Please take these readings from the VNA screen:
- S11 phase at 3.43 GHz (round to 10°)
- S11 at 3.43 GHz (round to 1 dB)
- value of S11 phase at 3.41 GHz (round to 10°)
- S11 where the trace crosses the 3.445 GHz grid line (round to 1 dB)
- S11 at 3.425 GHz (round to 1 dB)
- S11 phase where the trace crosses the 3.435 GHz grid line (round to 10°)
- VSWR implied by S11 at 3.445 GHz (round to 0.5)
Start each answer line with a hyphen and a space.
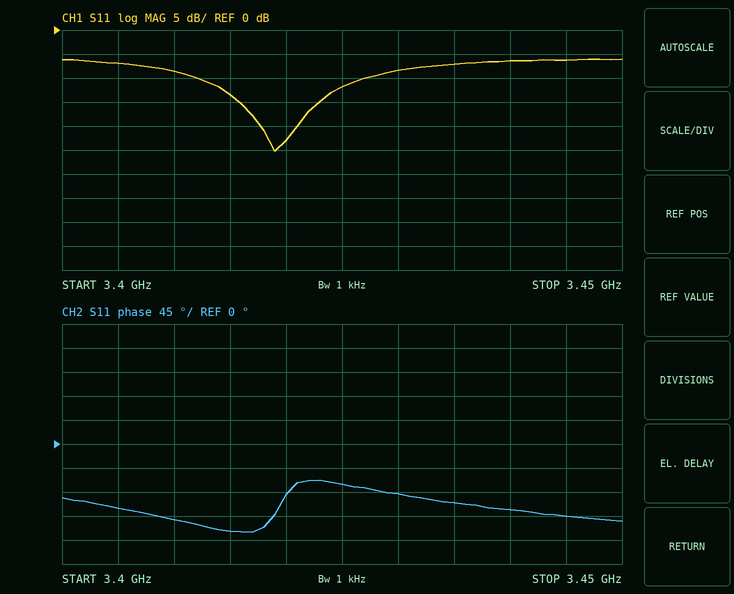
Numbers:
- -90°
- -8 dB
- -140°
- -6 dB
- -12 dB
- -110°
- 3.0
